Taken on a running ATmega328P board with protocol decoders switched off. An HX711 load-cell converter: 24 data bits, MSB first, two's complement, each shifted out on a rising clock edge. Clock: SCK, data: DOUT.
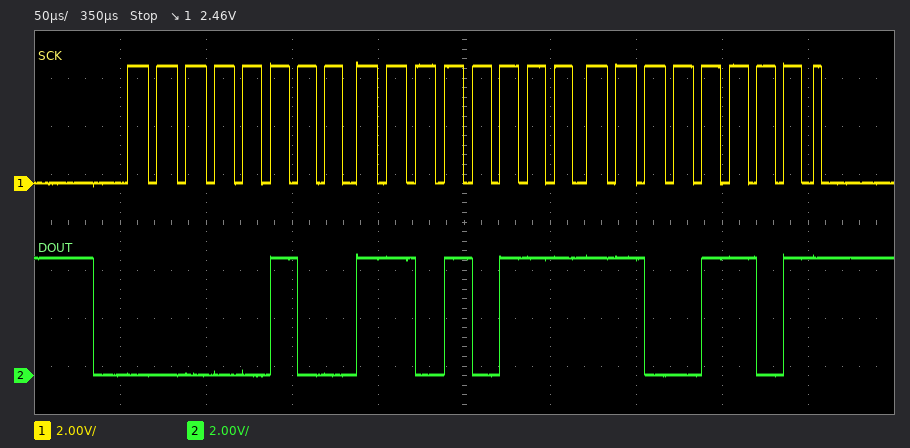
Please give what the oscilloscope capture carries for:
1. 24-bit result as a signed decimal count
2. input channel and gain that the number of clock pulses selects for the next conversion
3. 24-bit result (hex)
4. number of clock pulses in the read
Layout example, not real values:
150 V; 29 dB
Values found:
317389; channel A, gain 128; 0x04D7CD; 25
